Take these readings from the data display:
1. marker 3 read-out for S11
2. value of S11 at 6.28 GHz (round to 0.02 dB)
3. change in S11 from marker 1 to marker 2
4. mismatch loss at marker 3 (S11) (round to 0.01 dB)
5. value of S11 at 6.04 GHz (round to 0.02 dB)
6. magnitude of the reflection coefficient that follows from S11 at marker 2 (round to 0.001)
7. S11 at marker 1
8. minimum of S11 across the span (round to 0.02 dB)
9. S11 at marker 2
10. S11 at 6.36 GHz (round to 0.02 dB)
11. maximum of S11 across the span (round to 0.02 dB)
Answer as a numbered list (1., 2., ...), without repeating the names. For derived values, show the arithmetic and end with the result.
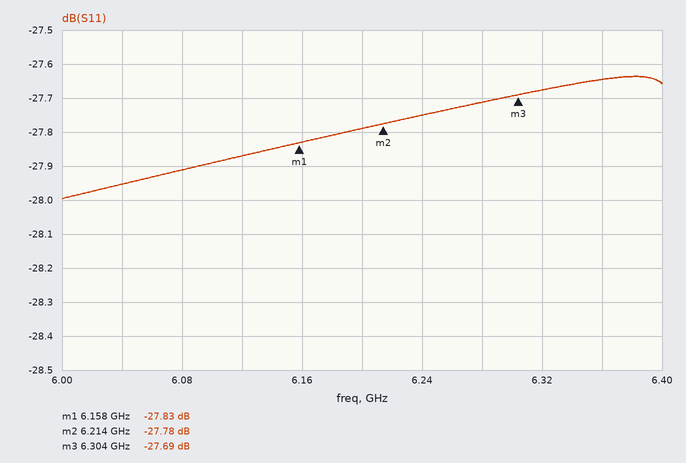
1. -27.69 dB
2. -27.72 dB
3. -27.78 − (-27.83) = 0.05 dB
4. −10 log10(1 − 10^(-27.69/10)) ≈ 0.01 dB
5. -27.96 dB
6. 10^(-27.78/20) ≈ 0.041
7. -27.83 dB
8. -28.00 dB
9. -27.78 dB
10. -27.64 dB
11. -27.64 dB
